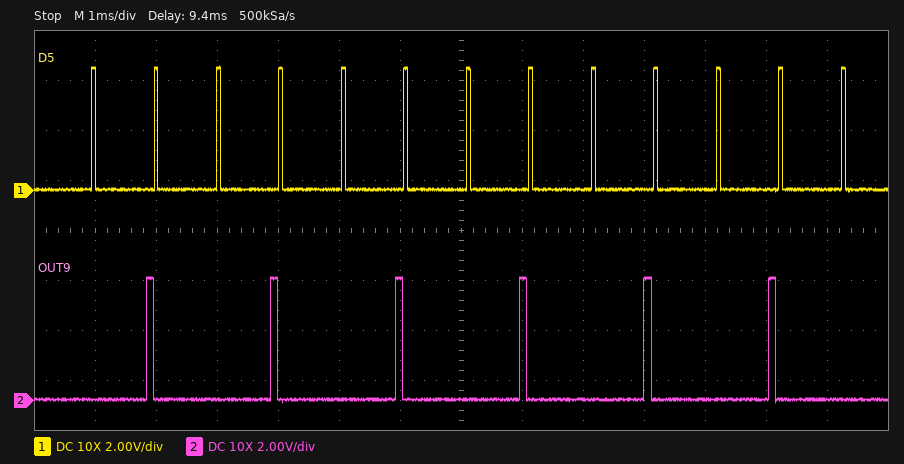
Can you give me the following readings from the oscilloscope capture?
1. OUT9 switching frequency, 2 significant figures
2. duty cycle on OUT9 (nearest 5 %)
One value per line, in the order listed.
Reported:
490 Hz
5 %
